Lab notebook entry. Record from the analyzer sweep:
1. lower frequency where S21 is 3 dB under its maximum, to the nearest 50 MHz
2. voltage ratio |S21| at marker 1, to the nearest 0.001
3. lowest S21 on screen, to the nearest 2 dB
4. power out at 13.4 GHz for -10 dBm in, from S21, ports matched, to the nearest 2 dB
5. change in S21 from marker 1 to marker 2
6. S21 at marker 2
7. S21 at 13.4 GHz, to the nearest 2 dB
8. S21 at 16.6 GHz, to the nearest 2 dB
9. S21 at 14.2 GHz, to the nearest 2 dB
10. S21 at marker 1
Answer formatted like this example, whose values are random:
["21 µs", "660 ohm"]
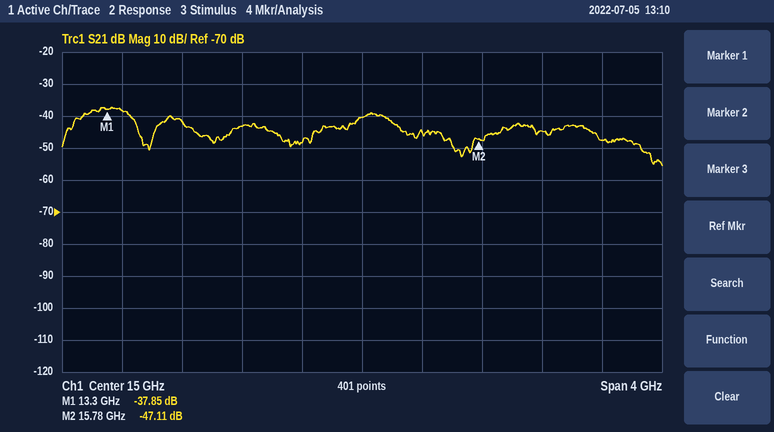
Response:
["13.15 GHz", "0.013", "-56 dB", "-48 dBm", "-9.26 dB", "-47.11 dB", "-38 dB", "-48 dB", "-44 dB", "-37.85 dB"]
